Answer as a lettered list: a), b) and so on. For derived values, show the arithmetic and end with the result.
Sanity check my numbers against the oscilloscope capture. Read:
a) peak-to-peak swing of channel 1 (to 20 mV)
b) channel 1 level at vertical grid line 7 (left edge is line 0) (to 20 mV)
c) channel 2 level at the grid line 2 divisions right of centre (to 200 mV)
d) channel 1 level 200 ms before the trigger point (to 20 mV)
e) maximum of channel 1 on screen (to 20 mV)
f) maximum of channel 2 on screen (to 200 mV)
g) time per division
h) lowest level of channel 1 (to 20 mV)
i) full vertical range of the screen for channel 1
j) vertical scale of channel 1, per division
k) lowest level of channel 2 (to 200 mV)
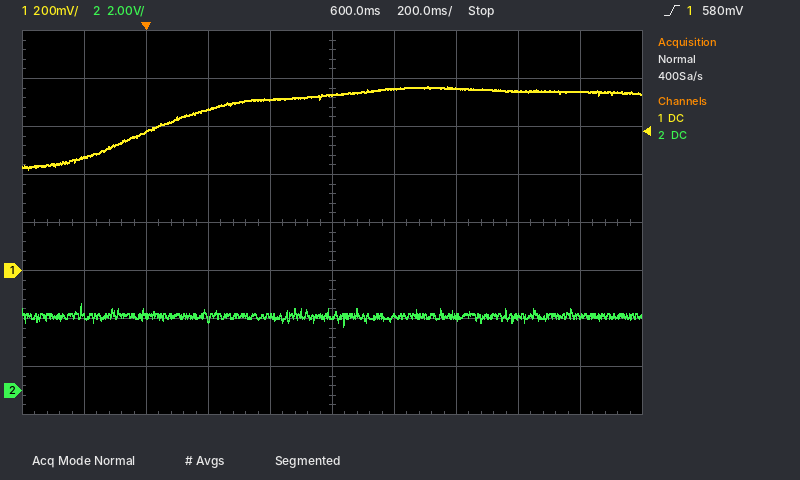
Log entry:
a) 760 mV − (420 mV) = 340 mV
b) 760 mV
c) 3.0 V
d) 480 mV
e) 760 mV
f) 3.6 V
g) 200 ms
h) 420 mV
i) 1.6 V
j) 200 mV
k) 2.6 V
